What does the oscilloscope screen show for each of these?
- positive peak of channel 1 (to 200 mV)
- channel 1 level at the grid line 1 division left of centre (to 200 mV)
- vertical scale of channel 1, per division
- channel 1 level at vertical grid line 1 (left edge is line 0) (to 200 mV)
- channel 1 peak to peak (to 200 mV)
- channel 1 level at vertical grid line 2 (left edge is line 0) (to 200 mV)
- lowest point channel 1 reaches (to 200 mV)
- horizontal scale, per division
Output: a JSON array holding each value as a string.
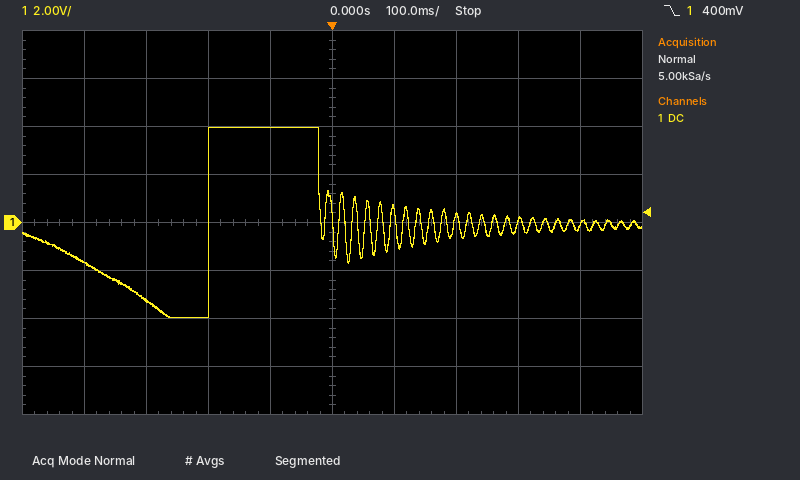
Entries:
["4.0 V", "4.0 V", "2 V", "-1.6 V", "8.0 V", "-3.2 V", "-4.0 V", "100 ms"]
